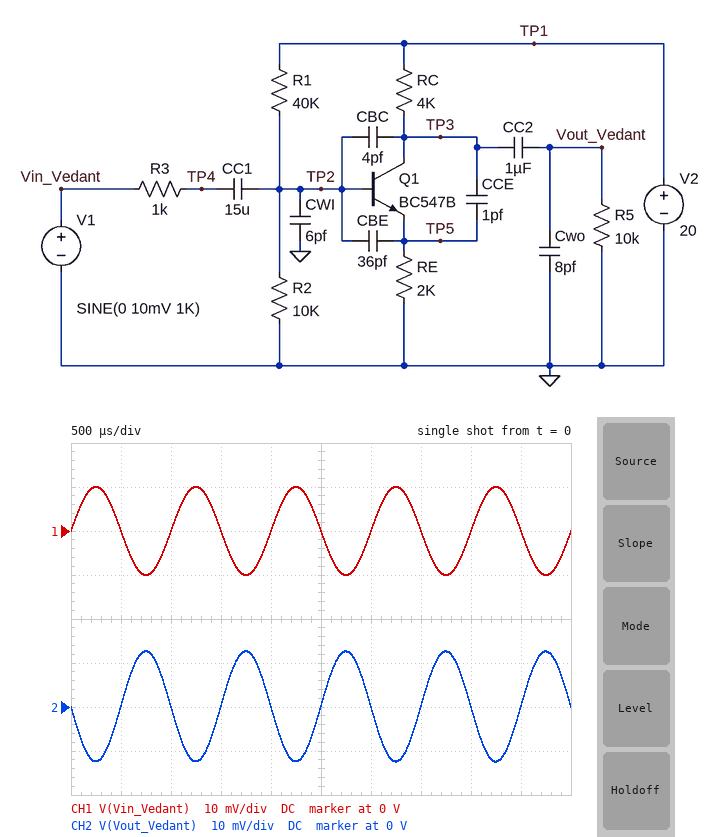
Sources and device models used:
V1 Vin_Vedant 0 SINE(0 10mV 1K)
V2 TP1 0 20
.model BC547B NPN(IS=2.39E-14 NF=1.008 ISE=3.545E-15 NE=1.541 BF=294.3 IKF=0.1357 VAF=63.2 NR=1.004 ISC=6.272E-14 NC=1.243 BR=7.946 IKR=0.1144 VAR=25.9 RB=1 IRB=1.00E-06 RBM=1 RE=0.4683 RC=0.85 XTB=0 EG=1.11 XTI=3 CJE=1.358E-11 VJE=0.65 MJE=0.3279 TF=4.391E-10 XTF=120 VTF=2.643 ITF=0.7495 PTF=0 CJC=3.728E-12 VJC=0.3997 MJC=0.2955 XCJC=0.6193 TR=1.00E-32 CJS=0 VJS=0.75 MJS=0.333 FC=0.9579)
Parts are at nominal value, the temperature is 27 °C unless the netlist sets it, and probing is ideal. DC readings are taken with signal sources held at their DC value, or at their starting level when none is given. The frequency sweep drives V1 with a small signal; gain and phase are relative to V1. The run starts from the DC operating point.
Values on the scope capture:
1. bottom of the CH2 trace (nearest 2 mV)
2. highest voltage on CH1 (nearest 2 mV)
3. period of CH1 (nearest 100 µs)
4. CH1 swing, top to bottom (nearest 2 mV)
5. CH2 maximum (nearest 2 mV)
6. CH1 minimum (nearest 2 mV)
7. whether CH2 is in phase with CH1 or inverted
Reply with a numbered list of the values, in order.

1. -12 mV
2. 10 mV
3. 1.0 ms
4. 20 mV
5. 12 mV
6. -10 mV
7. inverted
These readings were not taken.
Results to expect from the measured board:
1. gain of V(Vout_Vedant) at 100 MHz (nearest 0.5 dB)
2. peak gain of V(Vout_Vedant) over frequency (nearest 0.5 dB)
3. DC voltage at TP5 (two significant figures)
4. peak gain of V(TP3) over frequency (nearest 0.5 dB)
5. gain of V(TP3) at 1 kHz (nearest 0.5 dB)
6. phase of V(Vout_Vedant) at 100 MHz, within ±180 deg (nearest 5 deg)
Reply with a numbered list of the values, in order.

1. -22.5 dB
2. 2.0 dB
3. 3.3 V
4. 4.5 dB
5. 2.0 dB
6. -70 deg
